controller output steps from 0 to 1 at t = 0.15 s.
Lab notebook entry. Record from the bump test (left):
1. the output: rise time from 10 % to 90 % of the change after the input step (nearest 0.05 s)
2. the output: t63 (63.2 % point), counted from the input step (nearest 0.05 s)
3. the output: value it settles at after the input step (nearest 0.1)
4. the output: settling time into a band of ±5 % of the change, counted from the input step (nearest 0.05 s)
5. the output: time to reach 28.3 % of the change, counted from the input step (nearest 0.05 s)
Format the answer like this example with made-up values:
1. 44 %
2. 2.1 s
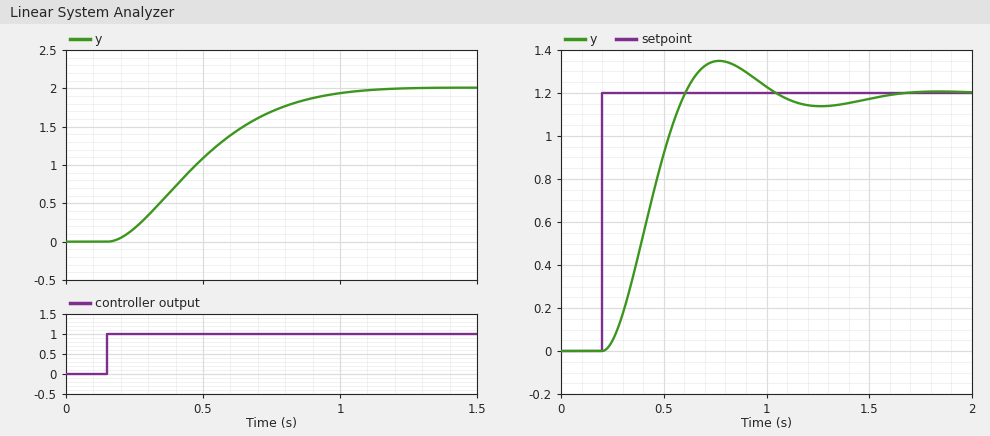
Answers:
1. 0.55 s
2. 0.40 s
3. 2.0
4. 0.80 s
5. 0.20 s
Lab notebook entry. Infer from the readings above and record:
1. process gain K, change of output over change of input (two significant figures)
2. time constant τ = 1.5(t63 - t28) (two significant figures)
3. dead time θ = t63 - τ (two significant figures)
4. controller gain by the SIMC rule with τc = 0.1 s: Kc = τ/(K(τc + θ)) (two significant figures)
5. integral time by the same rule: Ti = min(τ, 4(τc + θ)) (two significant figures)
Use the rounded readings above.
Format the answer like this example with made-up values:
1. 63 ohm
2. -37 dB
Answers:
1. 2.0
2. 0.30 s
3. 0.10 s
4. 0.75
5. 0.30 s
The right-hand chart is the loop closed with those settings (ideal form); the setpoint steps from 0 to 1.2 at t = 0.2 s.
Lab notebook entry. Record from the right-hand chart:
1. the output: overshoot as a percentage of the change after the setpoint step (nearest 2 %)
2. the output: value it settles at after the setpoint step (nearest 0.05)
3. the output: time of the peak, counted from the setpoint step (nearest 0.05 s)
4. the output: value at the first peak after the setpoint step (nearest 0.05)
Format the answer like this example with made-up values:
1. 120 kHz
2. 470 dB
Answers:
1. 12 %
2. 1.20
3. 0.55 s
4. 1.35
